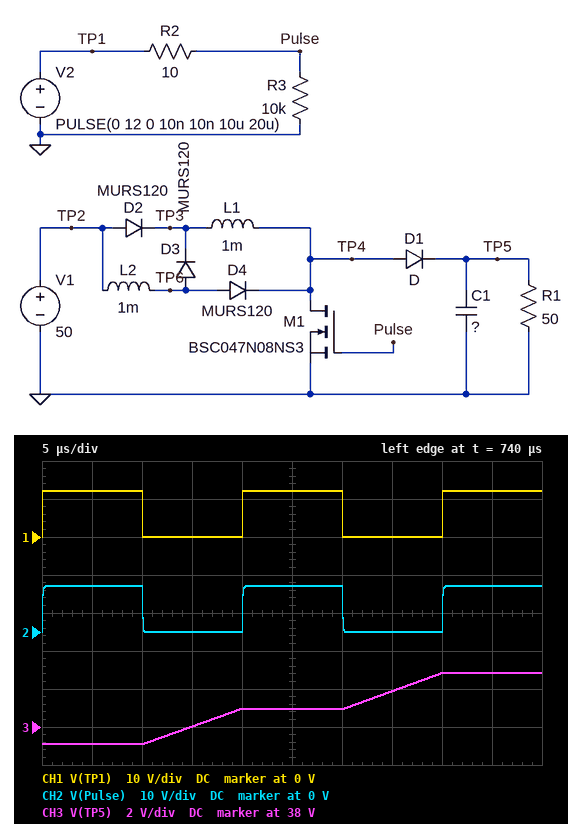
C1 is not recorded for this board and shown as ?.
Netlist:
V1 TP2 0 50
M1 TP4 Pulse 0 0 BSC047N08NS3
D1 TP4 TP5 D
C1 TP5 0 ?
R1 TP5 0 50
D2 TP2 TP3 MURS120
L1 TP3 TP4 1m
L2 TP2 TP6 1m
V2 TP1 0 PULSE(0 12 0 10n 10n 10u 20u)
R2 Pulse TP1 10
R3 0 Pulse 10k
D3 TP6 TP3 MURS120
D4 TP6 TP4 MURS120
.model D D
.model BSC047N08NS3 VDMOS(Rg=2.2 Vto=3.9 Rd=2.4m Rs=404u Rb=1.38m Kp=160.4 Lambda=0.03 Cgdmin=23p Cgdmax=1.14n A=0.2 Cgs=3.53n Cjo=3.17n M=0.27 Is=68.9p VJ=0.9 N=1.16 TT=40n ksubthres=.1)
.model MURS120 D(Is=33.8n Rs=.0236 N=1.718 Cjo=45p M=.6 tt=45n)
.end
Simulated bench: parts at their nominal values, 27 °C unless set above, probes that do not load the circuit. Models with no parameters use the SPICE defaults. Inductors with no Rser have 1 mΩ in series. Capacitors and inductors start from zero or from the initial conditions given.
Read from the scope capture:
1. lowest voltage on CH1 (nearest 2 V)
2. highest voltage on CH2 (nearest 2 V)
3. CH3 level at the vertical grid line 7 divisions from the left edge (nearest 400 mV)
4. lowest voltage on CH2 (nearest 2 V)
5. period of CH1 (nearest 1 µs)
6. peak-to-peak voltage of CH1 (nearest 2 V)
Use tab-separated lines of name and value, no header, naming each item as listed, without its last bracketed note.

lowest voltage on CH1	0 V
highest voltage on CH2	12 V
CH3 level at the vertical grid line 7 divisions from the left edge	40.0 V
lowest voltage on CH2	0 V
period of CH1	20 µs
peak-to-peak voltage of CH1	12 V
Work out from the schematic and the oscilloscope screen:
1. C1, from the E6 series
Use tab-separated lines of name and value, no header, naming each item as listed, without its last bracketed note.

C1, from the E6 series	330 µF
